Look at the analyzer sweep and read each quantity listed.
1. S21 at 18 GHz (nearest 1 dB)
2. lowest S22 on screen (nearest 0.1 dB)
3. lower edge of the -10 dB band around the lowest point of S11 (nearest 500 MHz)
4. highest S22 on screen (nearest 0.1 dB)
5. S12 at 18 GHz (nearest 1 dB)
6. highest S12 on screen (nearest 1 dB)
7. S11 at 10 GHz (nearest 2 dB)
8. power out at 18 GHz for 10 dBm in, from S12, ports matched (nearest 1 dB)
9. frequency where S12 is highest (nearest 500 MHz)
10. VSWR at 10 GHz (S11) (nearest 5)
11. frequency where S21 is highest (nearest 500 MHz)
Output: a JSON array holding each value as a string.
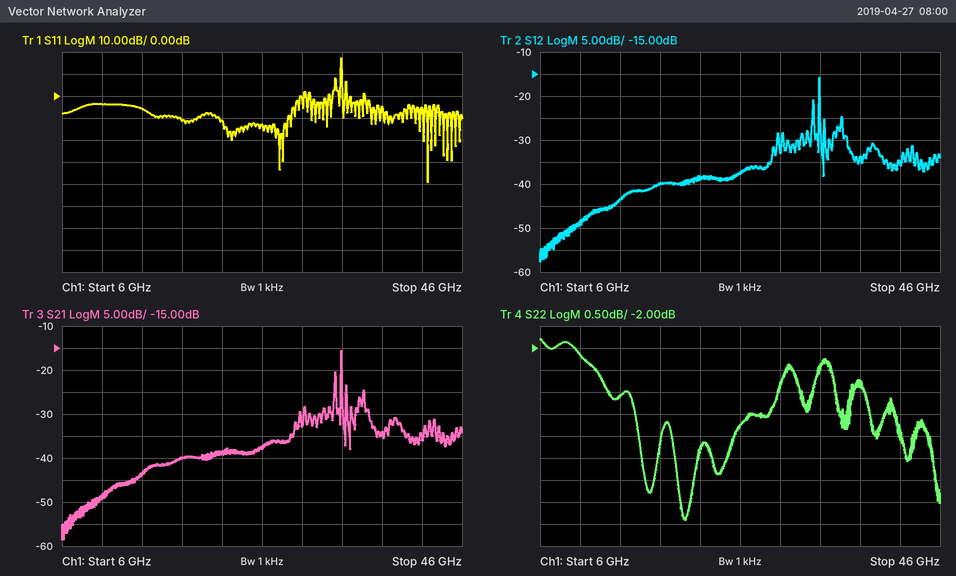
["-40 dB", "-5.9 dB", "42.5 GHz", "-1.8 dB", "-40 dB", "-16 dB", "-4 dB", "-30 dBm", "34.0 GHz", "5", "34.0 GHz"]
